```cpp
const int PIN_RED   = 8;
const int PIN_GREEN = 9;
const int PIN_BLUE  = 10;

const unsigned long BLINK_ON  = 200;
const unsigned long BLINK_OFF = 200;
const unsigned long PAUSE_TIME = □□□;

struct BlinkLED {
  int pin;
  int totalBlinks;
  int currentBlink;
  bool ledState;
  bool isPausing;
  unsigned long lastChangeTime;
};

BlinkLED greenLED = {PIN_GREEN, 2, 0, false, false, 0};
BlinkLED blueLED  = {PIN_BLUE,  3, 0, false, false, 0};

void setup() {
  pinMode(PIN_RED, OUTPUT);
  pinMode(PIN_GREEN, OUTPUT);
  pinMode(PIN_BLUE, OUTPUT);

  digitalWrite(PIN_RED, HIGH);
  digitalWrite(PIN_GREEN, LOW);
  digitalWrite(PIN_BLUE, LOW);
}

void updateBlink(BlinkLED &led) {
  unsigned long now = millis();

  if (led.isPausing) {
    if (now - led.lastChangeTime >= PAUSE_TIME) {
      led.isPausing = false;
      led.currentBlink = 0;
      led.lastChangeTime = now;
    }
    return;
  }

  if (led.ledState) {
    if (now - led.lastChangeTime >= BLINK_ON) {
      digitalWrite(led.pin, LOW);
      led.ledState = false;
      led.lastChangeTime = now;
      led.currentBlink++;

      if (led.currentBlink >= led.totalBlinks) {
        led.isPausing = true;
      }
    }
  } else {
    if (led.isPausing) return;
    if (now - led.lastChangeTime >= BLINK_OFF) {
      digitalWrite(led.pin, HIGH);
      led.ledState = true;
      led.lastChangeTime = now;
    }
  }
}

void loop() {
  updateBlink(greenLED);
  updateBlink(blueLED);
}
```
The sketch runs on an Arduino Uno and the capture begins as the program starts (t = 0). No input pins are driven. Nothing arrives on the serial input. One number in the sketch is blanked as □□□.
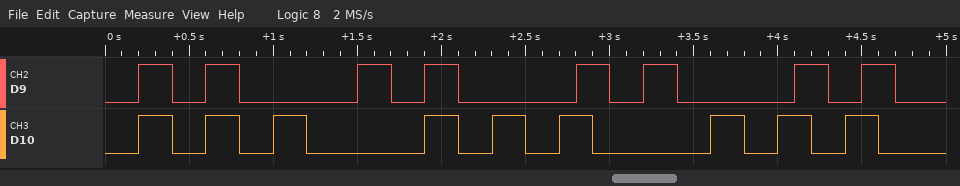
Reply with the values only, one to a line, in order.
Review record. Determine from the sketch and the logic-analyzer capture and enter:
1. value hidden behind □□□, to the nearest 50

500
